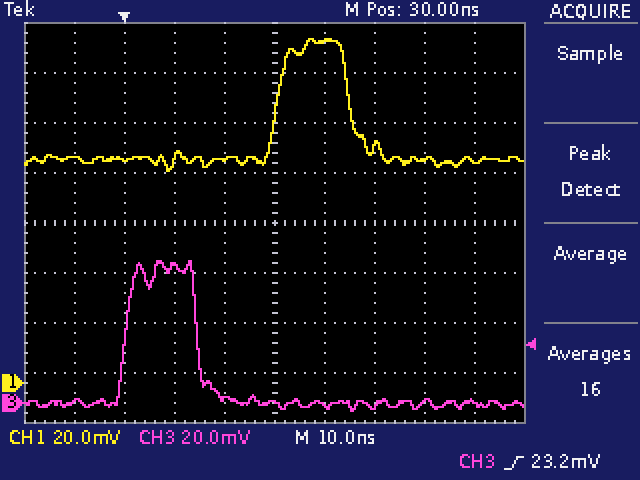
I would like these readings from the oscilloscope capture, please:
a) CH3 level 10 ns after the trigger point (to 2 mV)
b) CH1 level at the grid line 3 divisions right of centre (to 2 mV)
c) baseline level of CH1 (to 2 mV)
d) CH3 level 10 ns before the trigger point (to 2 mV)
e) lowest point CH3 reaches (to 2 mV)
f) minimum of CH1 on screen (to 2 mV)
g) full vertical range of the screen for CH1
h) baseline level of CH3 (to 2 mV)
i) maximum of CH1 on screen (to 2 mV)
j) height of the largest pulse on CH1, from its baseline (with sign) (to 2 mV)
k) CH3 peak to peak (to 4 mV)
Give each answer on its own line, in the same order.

54 mV
90 mV
90 mV
0 mV
-4 mV
84 mV
160 mV
0 mV
138 mV
+48 mV
60 mV
